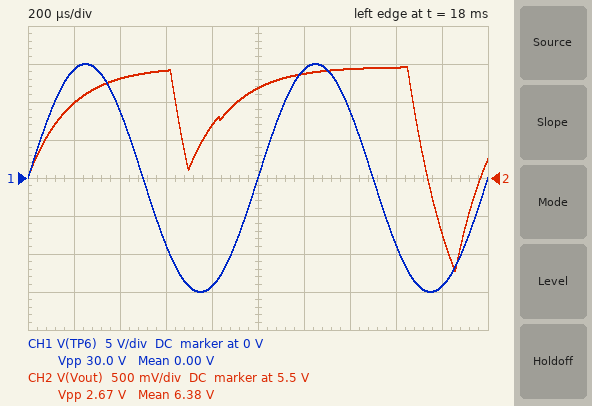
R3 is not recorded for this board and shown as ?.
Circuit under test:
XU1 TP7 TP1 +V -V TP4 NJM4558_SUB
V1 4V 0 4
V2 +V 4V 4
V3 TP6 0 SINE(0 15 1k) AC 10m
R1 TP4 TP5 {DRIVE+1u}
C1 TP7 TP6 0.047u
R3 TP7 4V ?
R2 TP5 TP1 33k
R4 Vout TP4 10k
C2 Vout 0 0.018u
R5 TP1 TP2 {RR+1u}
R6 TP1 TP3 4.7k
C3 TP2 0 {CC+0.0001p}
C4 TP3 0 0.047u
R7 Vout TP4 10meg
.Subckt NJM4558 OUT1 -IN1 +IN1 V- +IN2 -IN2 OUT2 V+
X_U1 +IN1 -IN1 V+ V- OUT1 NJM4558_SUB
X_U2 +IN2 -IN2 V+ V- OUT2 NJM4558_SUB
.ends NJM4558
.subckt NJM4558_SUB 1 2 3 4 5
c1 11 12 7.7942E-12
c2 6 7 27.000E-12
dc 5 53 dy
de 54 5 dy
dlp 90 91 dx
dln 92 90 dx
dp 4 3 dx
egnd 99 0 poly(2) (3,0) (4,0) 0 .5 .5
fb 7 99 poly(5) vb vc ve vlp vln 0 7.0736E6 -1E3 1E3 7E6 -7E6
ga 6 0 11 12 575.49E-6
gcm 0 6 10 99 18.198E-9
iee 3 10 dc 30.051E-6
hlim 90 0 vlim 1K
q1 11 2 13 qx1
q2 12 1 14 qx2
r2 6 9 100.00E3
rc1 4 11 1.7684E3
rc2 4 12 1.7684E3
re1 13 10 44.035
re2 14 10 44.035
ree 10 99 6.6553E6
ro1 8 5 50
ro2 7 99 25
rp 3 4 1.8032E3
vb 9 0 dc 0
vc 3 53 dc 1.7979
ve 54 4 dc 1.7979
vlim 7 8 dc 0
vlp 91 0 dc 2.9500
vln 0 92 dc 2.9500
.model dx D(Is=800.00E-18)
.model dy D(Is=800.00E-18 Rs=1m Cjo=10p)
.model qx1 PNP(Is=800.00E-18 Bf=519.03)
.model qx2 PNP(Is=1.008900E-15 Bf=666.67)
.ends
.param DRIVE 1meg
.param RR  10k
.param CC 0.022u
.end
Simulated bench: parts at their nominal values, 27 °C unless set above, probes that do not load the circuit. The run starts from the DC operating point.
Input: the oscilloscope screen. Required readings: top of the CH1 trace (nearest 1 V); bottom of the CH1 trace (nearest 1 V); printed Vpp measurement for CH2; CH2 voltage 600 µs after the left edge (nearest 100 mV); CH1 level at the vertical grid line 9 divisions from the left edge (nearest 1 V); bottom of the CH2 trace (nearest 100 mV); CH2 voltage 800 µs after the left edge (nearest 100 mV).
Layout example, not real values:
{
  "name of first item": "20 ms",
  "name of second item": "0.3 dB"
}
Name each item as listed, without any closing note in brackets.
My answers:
{
  "top of the CH1 trace": "15 V",
  "bottom of the CH1 trace": "-15 V",
  "printed Vpp measurement for CH2": "2.67 V",
  "CH2 voltage 600 µs after the left edge": "6.9 V",
  "CH1 level at the vertical grid line 9 divisions from the left edge": "-14 V",
  "bottom of the CH2 trace": "4.3 V",
  "CH2 voltage 800 µs after the left edge": "6.2 V"
}
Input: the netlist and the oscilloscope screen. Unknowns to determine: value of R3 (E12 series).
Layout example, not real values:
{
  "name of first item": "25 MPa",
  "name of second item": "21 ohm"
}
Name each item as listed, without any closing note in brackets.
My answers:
{
  "value of R3": "270 kΩ"
}
